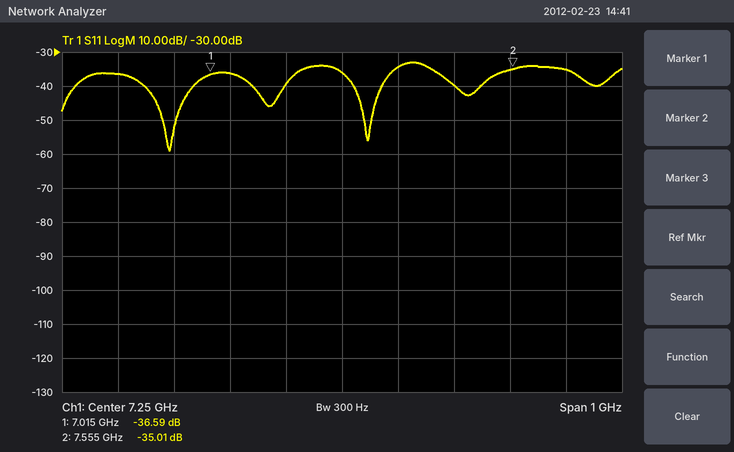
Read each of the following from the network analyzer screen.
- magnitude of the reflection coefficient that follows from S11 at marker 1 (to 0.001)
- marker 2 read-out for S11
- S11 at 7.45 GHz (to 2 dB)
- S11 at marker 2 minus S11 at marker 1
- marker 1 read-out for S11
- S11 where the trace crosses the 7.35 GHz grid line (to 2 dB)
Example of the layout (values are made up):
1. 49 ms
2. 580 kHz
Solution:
1. 0.015
2. -35.01 dB
3. -40 dB
4. 1.58 dB
5. -36.59 dB
6. -34 dB
